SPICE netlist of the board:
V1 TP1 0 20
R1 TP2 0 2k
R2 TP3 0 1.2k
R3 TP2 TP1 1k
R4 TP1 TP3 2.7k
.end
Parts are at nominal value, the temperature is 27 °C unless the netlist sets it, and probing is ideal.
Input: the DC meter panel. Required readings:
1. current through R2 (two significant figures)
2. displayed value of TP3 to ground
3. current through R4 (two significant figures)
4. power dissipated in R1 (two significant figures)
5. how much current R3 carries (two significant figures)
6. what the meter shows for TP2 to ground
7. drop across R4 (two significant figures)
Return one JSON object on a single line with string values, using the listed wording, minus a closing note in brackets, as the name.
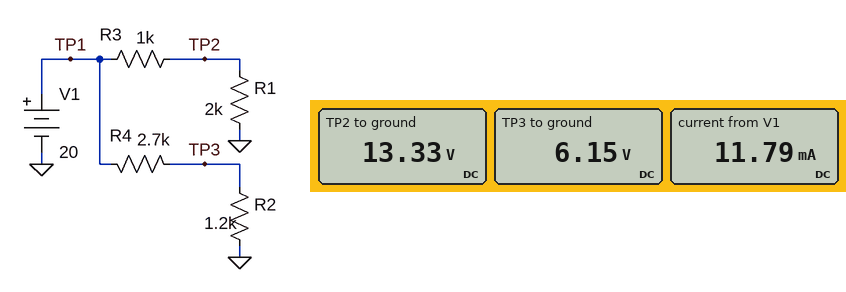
{"current through R2": "5.1 mA", "displayed value of TP3 to ground": "6.15 V", "current through R4": "5.1 mA", "power dissipated in R1": "89 mW", "how much current R3 carries": "6.7 mA", "what the meter shows for TP2 to ground": "13.33 V", "drop across R4": "14 V"}
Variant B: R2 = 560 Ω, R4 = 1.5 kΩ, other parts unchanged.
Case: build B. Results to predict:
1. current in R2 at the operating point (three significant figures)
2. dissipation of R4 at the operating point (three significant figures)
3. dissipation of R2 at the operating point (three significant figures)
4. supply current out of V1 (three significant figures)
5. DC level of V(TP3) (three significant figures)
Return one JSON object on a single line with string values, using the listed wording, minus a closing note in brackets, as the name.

{"current in R2 at the operating point": "9.71 mA", "dissipation of R4 at the operating point": "141 mW", "dissipation of R2 at the operating point": "52.8 mW", "supply current out of V1": "16.4 mA", "DC level of V(TP3)": "5.44 V"}
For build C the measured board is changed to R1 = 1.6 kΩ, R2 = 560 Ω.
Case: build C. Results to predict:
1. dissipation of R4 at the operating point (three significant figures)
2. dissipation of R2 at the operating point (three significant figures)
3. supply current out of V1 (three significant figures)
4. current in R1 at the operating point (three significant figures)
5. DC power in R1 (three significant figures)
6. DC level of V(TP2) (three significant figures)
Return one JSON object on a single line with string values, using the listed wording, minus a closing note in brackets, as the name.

{"dissipation of R4 at the operating point": "102 mW", "dissipation of R2 at the operating point": "21.1 mW", "supply current out of V1": "13.8 mA", "current in R1 at the operating point": "7.69 mA", "DC power in R1": "94.7 mW", "DC level of V(TP2)": "12.3 V"}
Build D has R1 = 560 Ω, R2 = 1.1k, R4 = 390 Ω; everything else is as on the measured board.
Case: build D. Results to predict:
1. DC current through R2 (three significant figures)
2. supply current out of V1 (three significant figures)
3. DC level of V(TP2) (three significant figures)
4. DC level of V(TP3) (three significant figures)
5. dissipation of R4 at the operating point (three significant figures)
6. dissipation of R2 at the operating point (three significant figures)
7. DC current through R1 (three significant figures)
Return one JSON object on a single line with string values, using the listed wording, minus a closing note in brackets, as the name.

{"DC current through R2": "13.4 mA", "supply current out of V1": "26.2 mA", "DC level of V(TP2)": "7.18 V", "DC level of V(TP3)": "14.8 V", "dissipation of R4 at the operating point": "70.3 mW", "dissipation of R2 at the operating point": "198 mW", "DC current through R1": "12.8 mA"}
